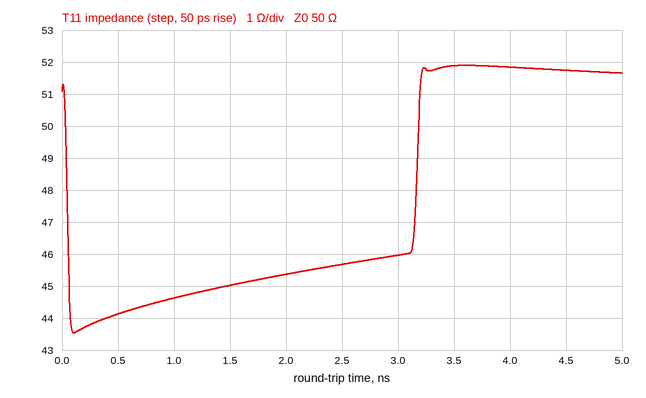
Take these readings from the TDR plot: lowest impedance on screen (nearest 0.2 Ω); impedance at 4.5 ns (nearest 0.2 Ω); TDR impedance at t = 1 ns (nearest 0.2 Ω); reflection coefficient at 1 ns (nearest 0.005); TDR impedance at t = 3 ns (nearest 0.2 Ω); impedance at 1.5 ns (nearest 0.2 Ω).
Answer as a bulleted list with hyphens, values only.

- 43.6 Ω
- 51.8 Ω
- 44.6 Ω
- -0.055
- 46.0 Ω
- 45.0 Ω
